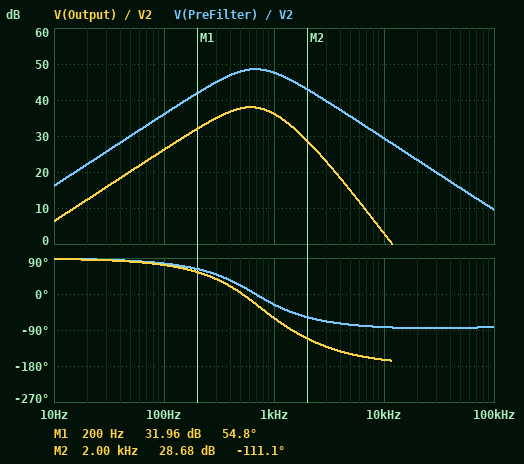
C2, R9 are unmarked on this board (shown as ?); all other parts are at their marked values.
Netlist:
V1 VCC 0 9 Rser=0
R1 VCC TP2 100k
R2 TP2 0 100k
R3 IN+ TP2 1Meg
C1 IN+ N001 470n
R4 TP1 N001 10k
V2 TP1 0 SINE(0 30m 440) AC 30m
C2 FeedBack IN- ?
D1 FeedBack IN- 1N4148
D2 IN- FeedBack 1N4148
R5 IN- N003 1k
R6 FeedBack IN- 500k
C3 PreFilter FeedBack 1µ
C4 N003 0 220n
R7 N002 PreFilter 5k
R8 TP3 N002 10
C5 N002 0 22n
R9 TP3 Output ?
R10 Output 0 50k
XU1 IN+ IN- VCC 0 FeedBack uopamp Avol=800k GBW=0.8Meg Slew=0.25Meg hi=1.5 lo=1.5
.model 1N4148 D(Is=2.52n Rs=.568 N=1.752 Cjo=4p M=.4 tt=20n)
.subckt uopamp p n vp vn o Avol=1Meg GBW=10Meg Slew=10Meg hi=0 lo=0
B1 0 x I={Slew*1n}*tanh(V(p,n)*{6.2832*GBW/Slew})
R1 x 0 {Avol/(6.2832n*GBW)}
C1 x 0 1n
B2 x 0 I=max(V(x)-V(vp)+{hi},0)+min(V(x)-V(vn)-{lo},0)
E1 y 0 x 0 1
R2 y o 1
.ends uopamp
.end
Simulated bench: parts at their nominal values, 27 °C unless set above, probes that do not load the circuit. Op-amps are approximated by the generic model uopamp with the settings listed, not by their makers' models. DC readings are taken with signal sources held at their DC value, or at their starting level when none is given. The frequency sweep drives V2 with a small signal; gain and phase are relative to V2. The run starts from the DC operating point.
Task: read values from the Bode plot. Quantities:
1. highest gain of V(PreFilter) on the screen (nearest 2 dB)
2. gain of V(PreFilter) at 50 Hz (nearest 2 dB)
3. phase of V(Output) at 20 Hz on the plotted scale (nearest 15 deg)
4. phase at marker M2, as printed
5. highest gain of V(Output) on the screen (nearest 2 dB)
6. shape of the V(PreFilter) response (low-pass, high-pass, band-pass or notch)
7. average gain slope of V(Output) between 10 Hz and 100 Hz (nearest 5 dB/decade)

48 dB
30 dB
90 deg
-111.1 deg
38 dB
band-pass
20 dB/decade
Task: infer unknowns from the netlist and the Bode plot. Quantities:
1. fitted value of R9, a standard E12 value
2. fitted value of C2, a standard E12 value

100 kΩ
330 pF
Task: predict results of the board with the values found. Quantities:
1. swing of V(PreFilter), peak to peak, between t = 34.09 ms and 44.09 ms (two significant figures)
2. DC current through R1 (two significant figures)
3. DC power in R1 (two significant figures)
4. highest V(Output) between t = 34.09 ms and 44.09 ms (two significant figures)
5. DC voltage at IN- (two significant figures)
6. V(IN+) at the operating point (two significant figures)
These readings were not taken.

810 mV
45 µA
200 µW
130 mV
4.5 V
4.5 V
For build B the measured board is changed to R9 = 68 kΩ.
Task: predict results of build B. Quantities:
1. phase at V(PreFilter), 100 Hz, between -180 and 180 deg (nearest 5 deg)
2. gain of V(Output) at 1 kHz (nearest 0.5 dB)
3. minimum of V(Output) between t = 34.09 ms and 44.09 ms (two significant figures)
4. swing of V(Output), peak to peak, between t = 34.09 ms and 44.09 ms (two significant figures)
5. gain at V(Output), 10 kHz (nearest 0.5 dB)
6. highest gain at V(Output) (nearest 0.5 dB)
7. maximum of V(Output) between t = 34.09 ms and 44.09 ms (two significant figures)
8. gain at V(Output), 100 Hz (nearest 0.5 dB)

75 deg
38.0 dB
-160 mV
330 mV
5.0 dB
40.0 dB
160 mV
28.0 dB
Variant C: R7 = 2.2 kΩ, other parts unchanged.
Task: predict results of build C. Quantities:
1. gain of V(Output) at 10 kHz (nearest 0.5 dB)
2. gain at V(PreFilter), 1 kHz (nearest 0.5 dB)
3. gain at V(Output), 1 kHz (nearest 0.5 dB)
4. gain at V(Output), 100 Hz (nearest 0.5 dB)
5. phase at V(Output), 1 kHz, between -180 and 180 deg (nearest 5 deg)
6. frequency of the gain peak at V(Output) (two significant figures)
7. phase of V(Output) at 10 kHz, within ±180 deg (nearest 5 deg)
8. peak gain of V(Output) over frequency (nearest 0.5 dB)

9.5 dB
47.5 dB
37.5 dB
26.5 dB
-45 deg
660 Hz
-155 deg
38.5 dB
